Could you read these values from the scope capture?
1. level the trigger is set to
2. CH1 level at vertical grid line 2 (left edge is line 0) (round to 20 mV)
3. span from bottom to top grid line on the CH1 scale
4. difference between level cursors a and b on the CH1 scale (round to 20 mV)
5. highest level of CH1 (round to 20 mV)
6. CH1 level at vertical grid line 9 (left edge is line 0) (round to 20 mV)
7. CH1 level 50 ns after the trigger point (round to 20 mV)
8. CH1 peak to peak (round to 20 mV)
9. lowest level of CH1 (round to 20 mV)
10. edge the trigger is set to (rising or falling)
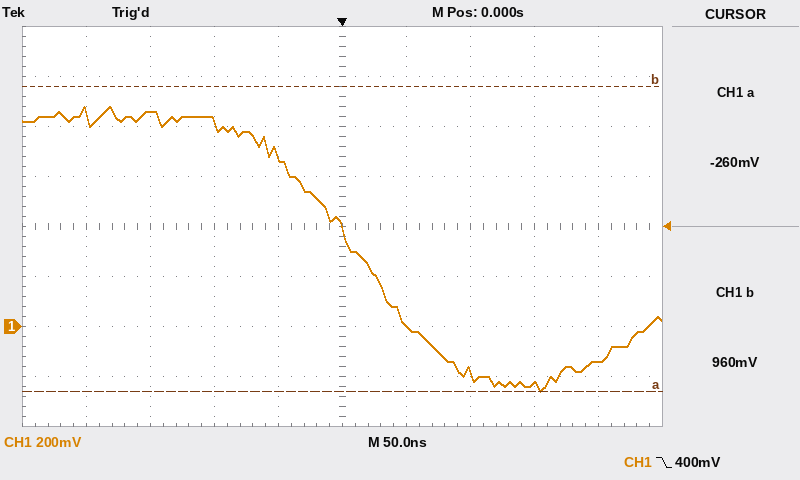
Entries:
400 mV
860 mV
1.6 V
1.22 V
880 mV
-140 mV
0 mV
1.14 V
-260 mV
falling
